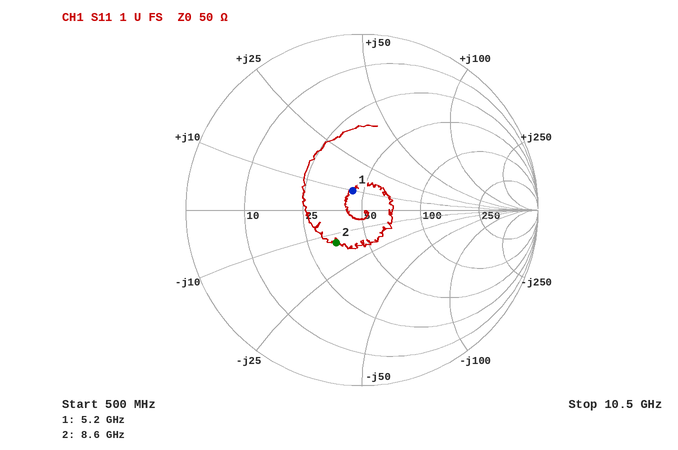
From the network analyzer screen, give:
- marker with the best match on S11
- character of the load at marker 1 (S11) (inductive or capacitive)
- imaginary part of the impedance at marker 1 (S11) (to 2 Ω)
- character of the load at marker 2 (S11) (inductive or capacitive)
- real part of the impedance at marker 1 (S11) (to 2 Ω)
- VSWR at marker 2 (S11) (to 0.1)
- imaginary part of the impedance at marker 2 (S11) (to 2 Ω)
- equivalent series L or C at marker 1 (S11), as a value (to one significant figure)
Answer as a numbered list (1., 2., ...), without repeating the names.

1. marker 1
2. inductive
3. +10 Ω
4. capacitive
5. 44 Ω
6. 1.6
7. -14 Ω
8. 300 pH
